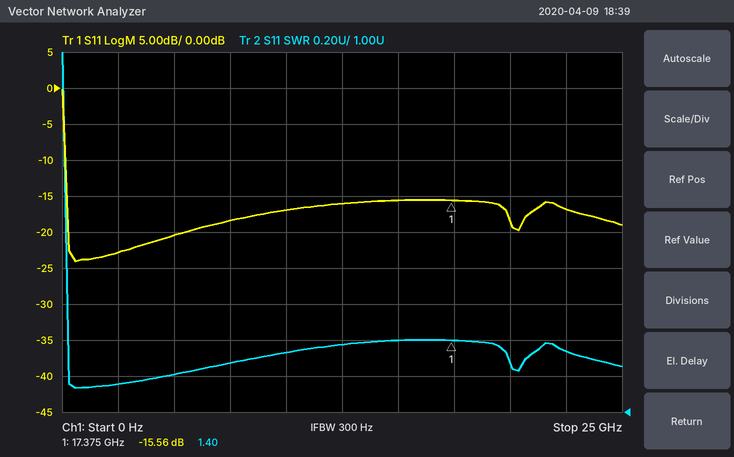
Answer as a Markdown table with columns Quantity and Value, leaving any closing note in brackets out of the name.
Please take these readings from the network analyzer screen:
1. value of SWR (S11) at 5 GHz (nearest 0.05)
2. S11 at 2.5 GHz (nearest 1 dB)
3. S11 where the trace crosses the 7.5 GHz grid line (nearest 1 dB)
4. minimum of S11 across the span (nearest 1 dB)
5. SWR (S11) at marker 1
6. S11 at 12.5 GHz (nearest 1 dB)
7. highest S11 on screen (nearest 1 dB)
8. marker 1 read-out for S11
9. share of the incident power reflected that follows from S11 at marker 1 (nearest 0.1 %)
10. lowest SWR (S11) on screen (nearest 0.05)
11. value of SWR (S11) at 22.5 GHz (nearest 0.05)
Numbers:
| Quantity | Value |
|---|---|
| value of SWR (S11) at 5 GHz | 1.20 |
| S11 at 2.5 GHz | -23 dB |
| S11 where the trace crosses the 7.5 GHz grid line | -18 dB |
| minimum of S11 across the span | -24 dB |
| SWR (S11) at marker 1 | 1.40 |
| S11 at 12.5 GHz | -16 dB |
| highest S11 on screen | 0 dB |
| marker 1 read-out for S11 | -15.56 dB |
| share of the incident power reflected that follows from S11 at marker 1 | 2.8 % |
| lowest SWR (S11) on screen | 1.15 |
| value of SWR (S11) at 22.5 GHz | 1.35 |
